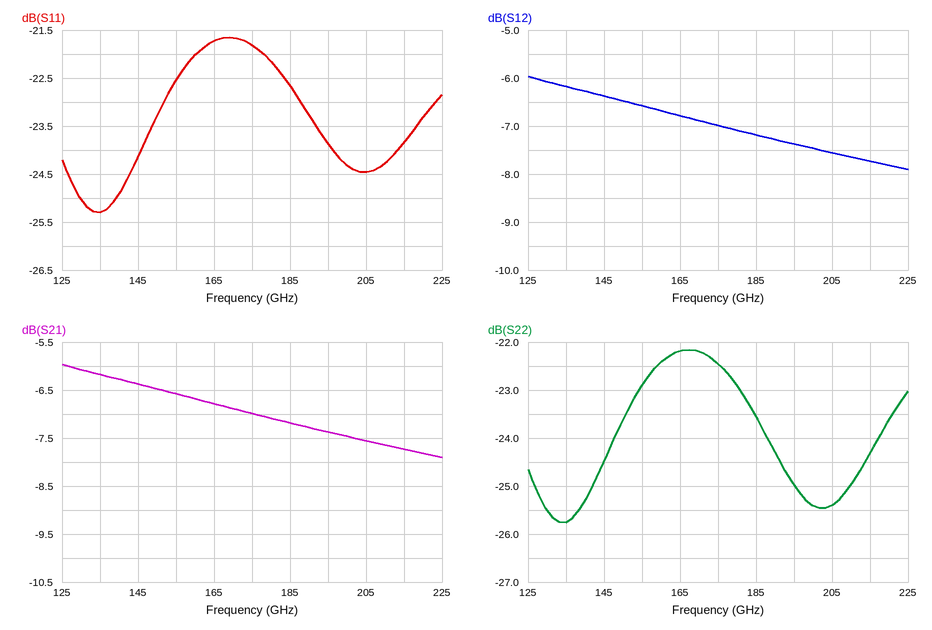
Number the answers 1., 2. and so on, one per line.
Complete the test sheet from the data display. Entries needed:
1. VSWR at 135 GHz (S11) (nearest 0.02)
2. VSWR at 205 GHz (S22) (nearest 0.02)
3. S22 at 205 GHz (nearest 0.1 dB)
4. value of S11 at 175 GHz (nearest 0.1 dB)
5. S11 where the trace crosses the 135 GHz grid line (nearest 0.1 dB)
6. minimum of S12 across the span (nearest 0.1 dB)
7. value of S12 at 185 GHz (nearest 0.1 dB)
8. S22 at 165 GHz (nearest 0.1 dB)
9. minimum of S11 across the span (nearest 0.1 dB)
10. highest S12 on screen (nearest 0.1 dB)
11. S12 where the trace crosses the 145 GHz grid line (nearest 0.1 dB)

1. 1.12
2. 1.12
3. -25.4 dB
4. -21.8 dB
5. -25.3 dB
6. -7.9 dB
7. -7.2 dB
8. -22.2 dB
9. -25.3 dB
10. -6.0 dB
11. -6.4 dB
